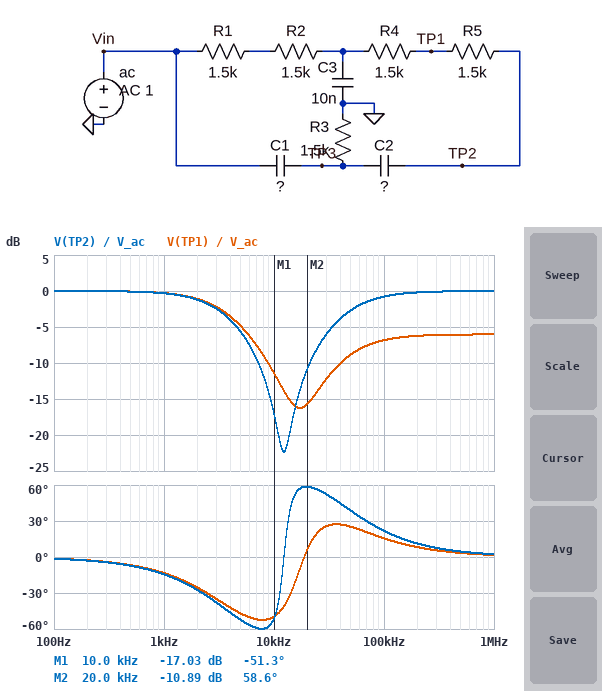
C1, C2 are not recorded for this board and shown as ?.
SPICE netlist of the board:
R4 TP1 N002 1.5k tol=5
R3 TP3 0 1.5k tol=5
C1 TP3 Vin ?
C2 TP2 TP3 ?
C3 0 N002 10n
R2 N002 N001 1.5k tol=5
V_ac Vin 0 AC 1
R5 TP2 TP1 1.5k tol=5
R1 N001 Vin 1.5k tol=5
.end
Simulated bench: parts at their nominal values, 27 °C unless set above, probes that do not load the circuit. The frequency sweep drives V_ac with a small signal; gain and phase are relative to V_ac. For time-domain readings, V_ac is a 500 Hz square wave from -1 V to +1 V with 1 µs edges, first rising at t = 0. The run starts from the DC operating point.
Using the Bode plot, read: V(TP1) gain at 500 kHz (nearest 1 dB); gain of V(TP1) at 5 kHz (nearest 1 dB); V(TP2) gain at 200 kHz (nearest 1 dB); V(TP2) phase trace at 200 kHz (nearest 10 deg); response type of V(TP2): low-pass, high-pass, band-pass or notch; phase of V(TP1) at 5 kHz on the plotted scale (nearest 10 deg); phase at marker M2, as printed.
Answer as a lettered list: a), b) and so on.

a) -6 dB
b) -5 dB
c) 0 dB
d) 10 deg
e) notch
f) -50 deg
g) 58.6 deg
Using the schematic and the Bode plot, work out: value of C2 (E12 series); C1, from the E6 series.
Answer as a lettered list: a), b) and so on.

a) 1.8 nF
b) 15 nF
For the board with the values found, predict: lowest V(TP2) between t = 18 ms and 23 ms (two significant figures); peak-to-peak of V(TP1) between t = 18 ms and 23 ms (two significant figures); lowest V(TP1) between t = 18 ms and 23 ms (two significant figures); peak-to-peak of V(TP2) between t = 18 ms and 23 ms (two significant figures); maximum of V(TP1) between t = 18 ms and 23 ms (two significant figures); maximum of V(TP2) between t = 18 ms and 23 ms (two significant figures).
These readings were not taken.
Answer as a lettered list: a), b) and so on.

a) -1.0 V
b) 2.0 V
c) -1.0 V
d) 2.0 V
e) 1.0 V
f) 1.0 V
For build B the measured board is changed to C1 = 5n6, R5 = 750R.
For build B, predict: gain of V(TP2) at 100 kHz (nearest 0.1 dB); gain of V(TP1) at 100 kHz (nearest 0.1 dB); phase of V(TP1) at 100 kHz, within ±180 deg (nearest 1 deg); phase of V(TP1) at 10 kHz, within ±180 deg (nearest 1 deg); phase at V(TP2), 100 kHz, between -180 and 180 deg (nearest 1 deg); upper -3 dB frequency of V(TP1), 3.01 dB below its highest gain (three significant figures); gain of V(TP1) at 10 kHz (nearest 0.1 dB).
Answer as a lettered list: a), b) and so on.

a) -1.8 dB
b) -5.4 dB
c) 33 deg
d) -69 deg
e) 36 deg
f) 3.95 kHz
g) -10.6 dB
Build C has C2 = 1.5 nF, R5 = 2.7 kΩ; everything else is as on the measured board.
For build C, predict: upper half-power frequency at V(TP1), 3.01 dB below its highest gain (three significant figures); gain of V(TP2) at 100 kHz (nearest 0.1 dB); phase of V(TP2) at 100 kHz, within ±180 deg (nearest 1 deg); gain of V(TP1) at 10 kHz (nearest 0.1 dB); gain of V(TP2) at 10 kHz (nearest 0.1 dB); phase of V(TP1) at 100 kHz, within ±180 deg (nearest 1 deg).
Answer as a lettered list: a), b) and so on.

a) 3.79 kHz
b) -0.6 dB
c) 19 deg
d) -10.4 dB
e) -19.5 dB
f) 10 deg
